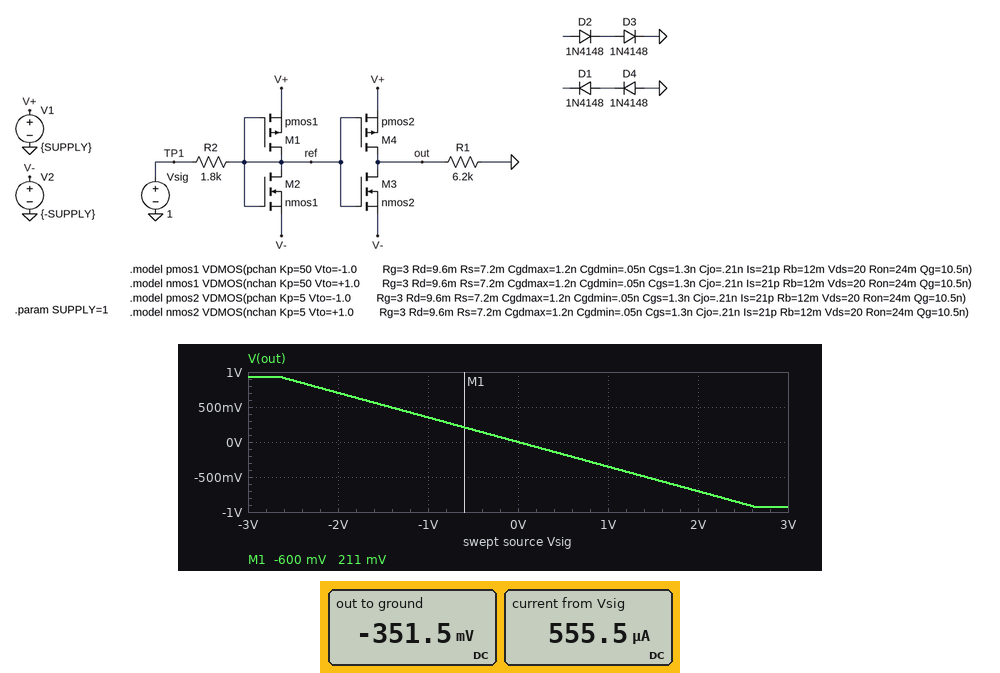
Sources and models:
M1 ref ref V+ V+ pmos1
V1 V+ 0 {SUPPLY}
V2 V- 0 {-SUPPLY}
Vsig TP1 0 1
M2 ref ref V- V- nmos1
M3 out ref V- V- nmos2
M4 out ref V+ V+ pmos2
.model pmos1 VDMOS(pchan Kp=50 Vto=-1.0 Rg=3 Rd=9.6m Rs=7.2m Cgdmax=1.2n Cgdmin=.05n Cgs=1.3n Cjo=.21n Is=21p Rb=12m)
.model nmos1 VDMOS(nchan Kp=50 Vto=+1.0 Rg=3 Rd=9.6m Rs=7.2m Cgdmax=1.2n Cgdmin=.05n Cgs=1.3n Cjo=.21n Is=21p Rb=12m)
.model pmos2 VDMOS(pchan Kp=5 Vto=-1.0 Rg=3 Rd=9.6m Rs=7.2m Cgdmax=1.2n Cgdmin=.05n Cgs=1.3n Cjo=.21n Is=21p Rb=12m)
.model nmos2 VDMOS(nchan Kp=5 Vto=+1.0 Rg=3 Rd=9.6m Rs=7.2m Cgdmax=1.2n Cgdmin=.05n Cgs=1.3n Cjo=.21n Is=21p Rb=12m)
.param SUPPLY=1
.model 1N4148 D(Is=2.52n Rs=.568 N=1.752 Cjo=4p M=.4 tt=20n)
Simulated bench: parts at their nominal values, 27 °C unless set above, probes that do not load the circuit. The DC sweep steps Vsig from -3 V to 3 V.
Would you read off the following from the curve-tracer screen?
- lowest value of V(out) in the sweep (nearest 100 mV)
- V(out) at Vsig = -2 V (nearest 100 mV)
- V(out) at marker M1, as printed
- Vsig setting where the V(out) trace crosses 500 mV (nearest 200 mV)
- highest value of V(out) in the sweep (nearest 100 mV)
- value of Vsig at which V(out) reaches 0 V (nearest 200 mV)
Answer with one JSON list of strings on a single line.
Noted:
["-900 mV", "700 mV", "211 mV", "-1.4 V", "900 mV", "0 V"]
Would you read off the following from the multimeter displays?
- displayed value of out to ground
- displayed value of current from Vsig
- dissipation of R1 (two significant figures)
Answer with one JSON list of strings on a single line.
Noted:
["-351.5 mV", "555.5 µA", "20 µW"]
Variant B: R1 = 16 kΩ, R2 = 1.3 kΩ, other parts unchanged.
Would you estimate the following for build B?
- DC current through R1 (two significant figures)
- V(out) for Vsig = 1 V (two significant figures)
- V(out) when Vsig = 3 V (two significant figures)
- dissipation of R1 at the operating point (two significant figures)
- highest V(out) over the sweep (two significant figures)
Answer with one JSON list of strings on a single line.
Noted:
["58 µA", "-930 mV", "-940 mV", "54 µW", "940 mV"]
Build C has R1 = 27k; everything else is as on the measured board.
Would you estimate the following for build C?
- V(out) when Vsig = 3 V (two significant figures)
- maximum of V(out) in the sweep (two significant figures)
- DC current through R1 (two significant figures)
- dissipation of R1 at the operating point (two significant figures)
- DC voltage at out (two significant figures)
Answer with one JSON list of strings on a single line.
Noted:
["-940 mV", "940 mV", "35 µA", "32 µW", "-930 mV"]
